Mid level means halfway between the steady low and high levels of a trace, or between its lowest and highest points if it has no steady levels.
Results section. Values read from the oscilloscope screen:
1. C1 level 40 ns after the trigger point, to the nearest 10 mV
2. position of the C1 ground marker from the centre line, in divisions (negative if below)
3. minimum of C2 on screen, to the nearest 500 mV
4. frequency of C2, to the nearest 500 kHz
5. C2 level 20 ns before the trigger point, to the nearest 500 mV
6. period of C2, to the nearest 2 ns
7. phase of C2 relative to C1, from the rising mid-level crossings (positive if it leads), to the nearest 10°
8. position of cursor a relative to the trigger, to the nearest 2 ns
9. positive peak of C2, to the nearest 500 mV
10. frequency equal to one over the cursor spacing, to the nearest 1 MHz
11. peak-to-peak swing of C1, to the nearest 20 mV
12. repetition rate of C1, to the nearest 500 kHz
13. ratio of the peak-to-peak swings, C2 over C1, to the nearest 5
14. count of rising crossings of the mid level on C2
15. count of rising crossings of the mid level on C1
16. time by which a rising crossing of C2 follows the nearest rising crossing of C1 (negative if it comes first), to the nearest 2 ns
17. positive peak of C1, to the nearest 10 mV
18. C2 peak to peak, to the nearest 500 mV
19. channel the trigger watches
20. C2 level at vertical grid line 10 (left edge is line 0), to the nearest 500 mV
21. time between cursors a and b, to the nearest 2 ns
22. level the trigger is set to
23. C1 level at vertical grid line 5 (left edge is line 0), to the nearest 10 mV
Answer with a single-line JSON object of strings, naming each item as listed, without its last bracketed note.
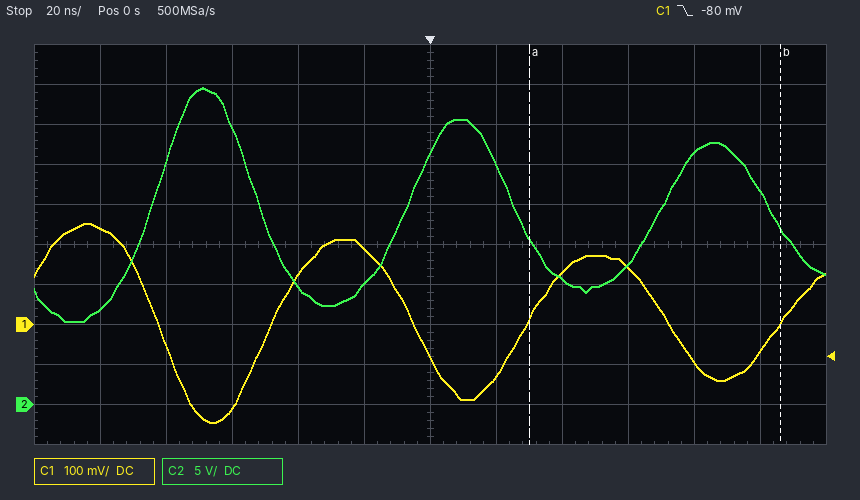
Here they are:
{"C1 level 40 ns after the trigger point, to the nearest 10 mV": "130 mV", "position of the C1 ground marker from the centre line, in divisions": "-2.0 div", "minimum of C2 on screen, to the nearest 500 mV": "10.5 V", "frequency of C2, to the nearest 500 kHz": "13.0 MHz", "C2 level 20 ns before the trigger point, to the nearest 500 mV": "15.0 V", "period of C2, to the nearest 2 ns": "78 ns", "phase of C2 relative to C1, from the rising mid-level crossings (positive if it leads), to the nearest 10°": "+170°", "position of cursor a relative to the trigger, to the nearest 2 ns": "+30 ns", "positive peak of C2, to the nearest 500 mV": "39.5 V", "frequency equal to one over the cursor spacing, to the nearest 1 MHz": "13 MHz", "peak-to-peak swing of C1, to the nearest 20 mV": "500 mV", "repetition rate of C1, to the nearest 500 kHz": "13.0 MHz", "ratio of the peak-to-peak swings, C2 over C1, to the nearest 5": "60", "count of rising crossings of the mid level on C2": "3", "count of rising crossings of the mid level on C1": "3", "time by which a rising crossing of C2 follows the nearest rising crossing of C1 (negative if it comes first), to the nearest 2 ns": "-36 ns", "positive peak of C1, to the nearest 10 mV": "250 mV", "C2 peak to peak, to the nearest 500 mV": "29.0 V", "channel the trigger watches": "C1", "C2 level at vertical grid line 10 (left edge is line 0), to the nearest 500 mV": "31.5 V", "time between cursors a and b, to the nearest 2 ns": "76 ns", "level the trigger is set to": "-80 mV", "C1 level at vertical grid line 5 (left edge is line 0), to the nearest 10 mV": "190 mV"}
